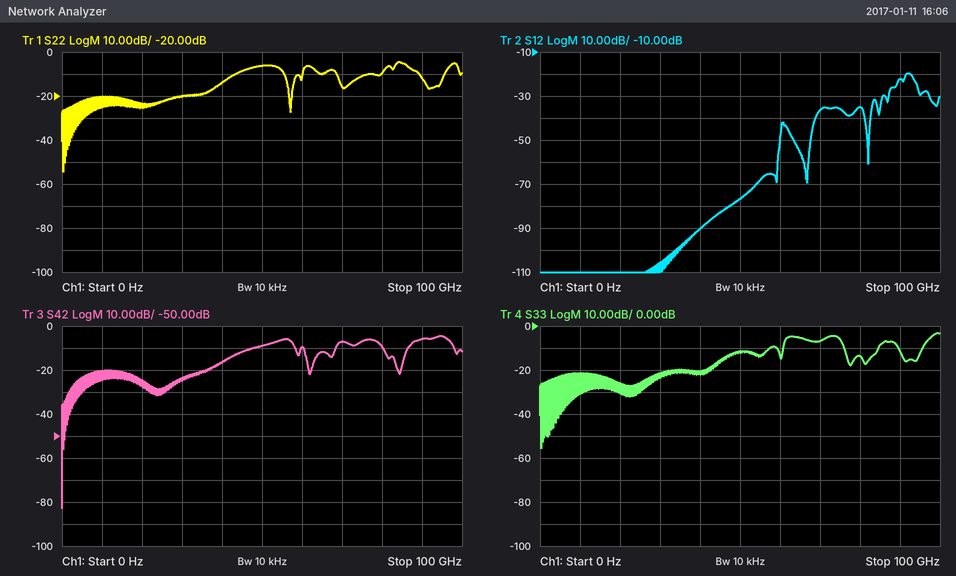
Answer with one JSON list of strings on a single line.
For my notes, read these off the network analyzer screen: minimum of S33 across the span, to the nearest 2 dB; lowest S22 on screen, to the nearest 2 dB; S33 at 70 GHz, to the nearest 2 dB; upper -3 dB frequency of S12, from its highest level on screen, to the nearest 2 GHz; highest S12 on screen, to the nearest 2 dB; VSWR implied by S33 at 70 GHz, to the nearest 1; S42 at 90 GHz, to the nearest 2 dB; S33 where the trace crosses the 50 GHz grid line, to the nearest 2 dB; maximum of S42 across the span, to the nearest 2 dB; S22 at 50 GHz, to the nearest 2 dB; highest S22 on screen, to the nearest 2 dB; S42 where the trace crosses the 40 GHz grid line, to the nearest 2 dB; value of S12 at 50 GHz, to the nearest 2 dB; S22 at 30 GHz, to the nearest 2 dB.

["-56 dB", "-54 dB", "-6 dB", "94 GHz", "-20 dB", "3", "-6 dB", "-12 dB", "-4 dB", "-6 dB", "-4 dB", "-16 dB", "-76 dB", "-20 dB"]
